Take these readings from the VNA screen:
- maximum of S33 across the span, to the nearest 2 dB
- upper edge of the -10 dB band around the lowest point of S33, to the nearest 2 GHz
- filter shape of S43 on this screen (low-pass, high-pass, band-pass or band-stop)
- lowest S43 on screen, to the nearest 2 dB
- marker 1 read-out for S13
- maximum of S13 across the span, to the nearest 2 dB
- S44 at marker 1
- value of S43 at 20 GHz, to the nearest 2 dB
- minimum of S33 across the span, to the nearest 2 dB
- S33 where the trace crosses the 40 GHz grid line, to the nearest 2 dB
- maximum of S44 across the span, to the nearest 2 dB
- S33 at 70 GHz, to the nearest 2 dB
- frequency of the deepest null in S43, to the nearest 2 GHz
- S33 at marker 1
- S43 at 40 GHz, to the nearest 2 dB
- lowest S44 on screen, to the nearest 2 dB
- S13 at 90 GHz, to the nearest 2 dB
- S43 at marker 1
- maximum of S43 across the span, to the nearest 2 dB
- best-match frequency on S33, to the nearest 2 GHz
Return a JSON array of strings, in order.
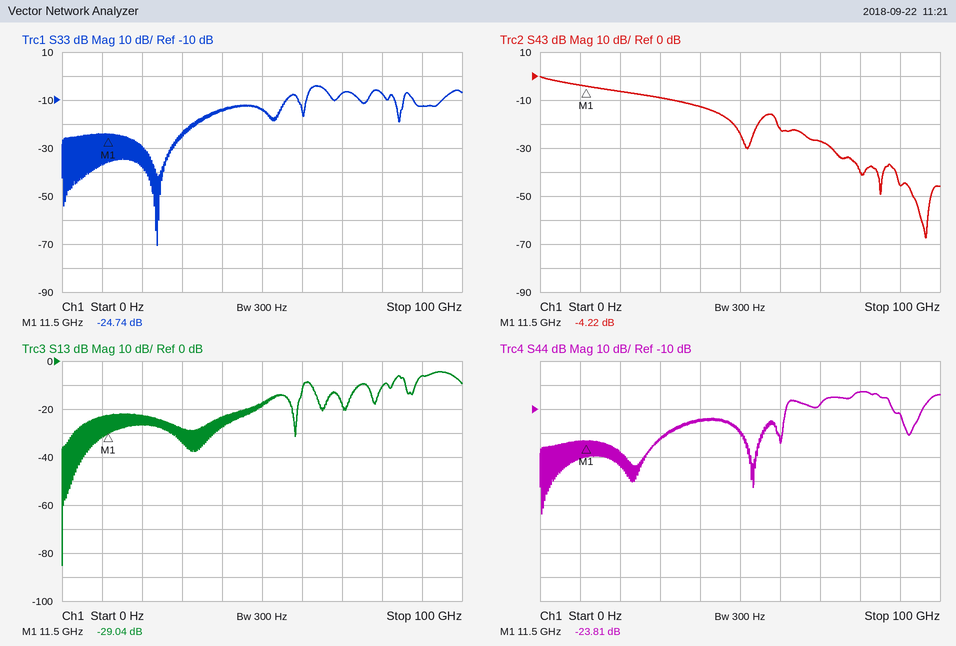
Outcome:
["-4 dB", "56 GHz", "low-pass", "-68 dB", "-29.04 dB", "-4 dB", "-23.81 dB", "-6 dB", "-70 dB", "-14 dB", "-2 dB", "-8 dB", "96 GHz", "-24.74 dB", "-12 dB", "-54 dB", "-6 dB", "-4.22 dB", "0 dB", "24 GHz"]
